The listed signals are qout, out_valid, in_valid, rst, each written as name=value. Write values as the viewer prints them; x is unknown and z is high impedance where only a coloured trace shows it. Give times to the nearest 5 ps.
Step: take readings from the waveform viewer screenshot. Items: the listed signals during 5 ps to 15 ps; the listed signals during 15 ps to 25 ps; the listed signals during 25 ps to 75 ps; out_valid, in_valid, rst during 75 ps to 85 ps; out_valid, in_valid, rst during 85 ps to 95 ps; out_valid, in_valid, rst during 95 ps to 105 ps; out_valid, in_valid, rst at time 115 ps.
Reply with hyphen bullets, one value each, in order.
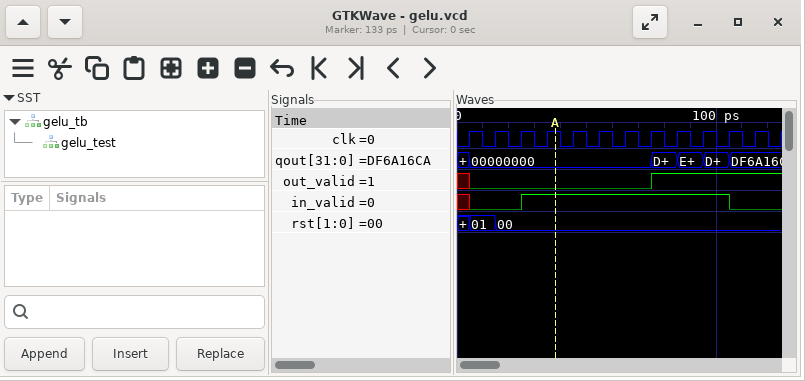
- qout=00000000, out_valid=0, in_valid=0, rst=01
- qout=00000000, out_valid=0, in_valid=0, rst=00
- qout=00000000, out_valid=0, in_valid=1, rst=00
- out_valid=1, in_valid=1, rst=00
- out_valid=1, in_valid=1, rst=00
- out_valid=1, in_valid=1, rst=00
- out_valid=1, in_valid=0, rst=00
